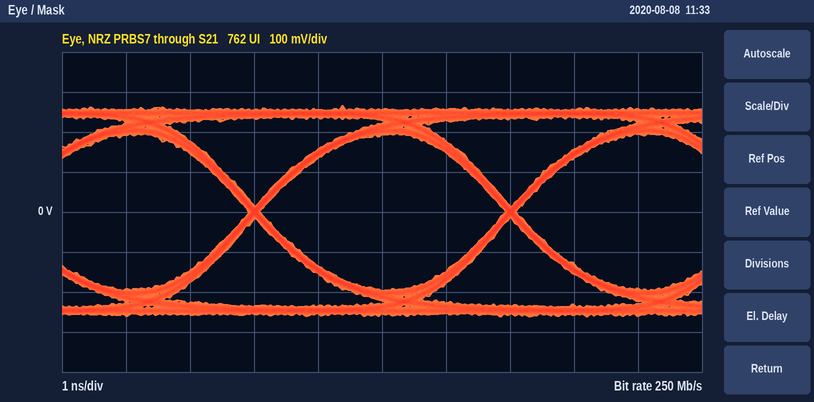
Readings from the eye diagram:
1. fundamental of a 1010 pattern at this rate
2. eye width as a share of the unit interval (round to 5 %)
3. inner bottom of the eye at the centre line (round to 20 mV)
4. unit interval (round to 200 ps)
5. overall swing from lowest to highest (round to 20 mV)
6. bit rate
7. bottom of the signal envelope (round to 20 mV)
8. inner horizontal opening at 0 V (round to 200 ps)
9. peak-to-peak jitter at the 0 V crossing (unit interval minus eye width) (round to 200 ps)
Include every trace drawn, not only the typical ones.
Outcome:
125 MHz
95 %
-200 mV
4.0 ns
520 mV
250 Mb/s
-260 mV
3.8 ns
200 ps
